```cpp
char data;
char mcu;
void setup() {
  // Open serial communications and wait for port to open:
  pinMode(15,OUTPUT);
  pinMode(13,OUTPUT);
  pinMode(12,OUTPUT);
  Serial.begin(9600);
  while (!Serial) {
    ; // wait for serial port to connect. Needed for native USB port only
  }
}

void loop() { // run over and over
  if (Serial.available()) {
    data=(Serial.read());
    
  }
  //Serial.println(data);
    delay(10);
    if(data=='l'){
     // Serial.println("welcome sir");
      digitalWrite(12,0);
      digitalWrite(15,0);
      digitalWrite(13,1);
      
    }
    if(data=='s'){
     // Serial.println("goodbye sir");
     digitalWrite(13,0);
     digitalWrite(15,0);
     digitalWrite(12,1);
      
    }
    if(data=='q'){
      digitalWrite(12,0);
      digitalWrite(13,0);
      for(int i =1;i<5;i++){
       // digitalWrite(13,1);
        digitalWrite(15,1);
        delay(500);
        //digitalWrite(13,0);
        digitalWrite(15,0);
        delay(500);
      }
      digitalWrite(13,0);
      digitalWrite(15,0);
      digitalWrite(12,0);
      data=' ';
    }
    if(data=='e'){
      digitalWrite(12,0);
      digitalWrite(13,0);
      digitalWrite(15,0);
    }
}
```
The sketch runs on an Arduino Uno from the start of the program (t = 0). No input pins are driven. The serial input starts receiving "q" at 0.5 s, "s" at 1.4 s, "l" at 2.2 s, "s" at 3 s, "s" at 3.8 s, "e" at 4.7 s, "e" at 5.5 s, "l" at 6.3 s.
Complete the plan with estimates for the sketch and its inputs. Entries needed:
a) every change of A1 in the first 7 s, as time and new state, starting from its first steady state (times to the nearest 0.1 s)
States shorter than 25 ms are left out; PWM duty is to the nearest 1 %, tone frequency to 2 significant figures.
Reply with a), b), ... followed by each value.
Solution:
a) 0 s low; 0.5 s high; 1 s low; 1.5 s high; 2 s low; 2.5 s high; 3 s low; 3.5 s high; 4 s low
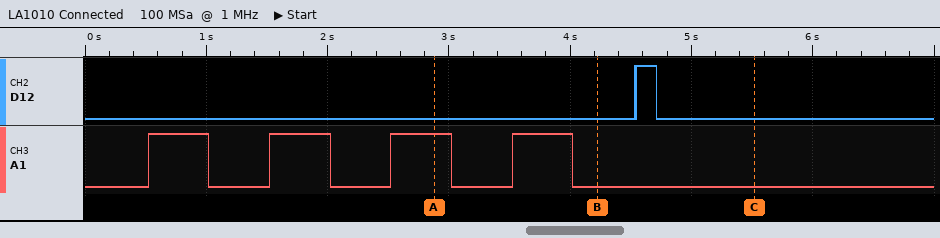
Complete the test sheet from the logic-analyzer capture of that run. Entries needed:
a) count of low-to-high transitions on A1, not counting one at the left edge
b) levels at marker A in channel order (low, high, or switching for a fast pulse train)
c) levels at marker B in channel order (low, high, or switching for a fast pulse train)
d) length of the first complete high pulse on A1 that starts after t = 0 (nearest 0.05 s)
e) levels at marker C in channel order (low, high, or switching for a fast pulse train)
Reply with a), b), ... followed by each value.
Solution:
a) 4
b) D12 low, A1 high
c) D12 low, A1 low
d) 0.50 s
e) D12 low, A1 low
